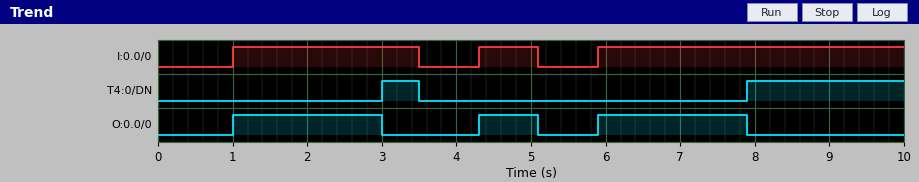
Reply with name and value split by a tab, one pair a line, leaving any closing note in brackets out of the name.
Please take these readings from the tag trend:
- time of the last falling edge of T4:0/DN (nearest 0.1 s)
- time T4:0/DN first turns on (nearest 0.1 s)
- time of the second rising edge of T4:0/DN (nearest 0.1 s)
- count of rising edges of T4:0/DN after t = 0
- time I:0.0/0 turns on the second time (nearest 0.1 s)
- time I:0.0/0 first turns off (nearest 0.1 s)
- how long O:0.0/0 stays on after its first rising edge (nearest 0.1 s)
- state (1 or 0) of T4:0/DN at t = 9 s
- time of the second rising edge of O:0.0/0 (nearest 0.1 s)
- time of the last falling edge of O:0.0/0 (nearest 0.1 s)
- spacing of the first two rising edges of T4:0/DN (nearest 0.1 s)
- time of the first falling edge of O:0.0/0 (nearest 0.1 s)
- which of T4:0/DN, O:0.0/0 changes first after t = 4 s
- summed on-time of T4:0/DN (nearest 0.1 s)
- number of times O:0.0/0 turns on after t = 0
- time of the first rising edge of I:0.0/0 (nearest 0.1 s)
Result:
time of the last falling edge of T4:0/DN	3.5 s
time T4:0/DN first turns on	3.0 s
time of the second rising edge of T4:0/DN	7.9 s
count of rising edges of T4:0/DN after t = 0	2
time I:0.0/0 turns on the second time	4.3 s
time I:0.0/0 first turns off	3.5 s
how long O:0.0/0 stays on after its first rising edge	2.0 s
state (1 or 0) of T4:0/DN at t = 9 s	1
time of the second rising edge of O:0.0/0	4.3 s
time of the last falling edge of O:0.0/0	7.9 s
spacing of the first two rising edges of T4:0/DN	4.9 s
time of the first falling edge of O:0.0/0	3.0 s
which of T4:0/DN, O:0.0/0 changes first after t = 4 s	O:0.0/0
summed on-time of T4:0/DN	2.6 s
number of times O:0.0/0 turns on after t = 0	3
time of the first rising edge of I:0.0/0	1.0 s
